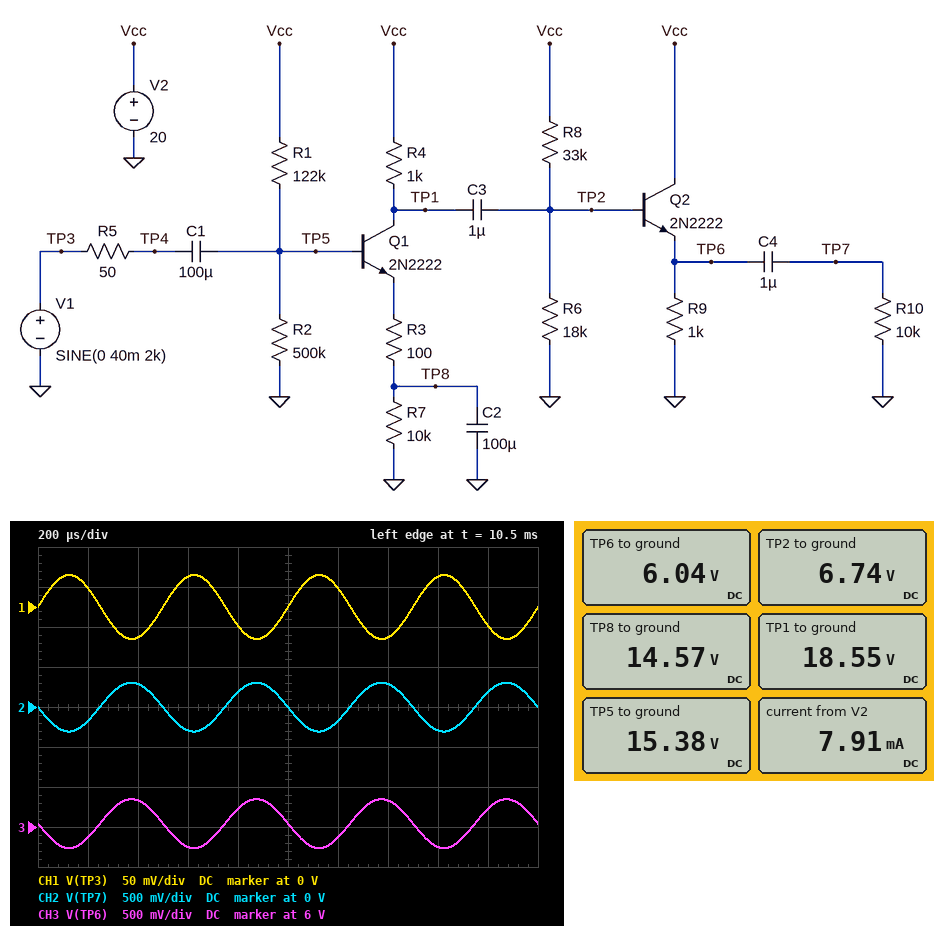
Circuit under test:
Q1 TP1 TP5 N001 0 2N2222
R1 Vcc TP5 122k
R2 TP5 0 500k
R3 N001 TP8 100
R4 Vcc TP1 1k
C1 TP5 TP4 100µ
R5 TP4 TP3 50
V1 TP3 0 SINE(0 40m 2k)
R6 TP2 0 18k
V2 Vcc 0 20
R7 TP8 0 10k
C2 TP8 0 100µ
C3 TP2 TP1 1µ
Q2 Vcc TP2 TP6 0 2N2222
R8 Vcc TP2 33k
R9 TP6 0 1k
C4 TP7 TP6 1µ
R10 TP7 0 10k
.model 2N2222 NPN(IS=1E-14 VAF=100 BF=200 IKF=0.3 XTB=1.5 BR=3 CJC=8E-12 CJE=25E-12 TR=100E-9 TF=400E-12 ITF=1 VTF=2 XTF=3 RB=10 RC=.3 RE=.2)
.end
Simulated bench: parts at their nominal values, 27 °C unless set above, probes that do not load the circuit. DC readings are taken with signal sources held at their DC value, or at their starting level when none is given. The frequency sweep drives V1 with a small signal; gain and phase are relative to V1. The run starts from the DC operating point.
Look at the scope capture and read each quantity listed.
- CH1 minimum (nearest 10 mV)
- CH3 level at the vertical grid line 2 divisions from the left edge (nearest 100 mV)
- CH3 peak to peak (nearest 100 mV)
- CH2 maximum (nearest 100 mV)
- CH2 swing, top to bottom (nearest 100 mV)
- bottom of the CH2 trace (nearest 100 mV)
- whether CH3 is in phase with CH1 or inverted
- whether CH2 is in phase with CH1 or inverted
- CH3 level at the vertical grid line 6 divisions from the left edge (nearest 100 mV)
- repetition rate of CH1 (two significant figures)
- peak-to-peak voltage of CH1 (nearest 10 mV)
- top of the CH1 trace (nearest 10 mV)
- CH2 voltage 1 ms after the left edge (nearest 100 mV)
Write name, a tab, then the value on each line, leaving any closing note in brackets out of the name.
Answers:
CH1 minimum	-40 mV
CH3 level at the vertical grid line 2 divisions from the left edge	6.3 V
CH3 peak to peak	600 mV
CH2 maximum	300 mV
CH2 swing, top to bottom	600 mV
bottom of the CH2 trace	-300 mV
whether CH3 is in phase with CH1 or inverted	inverted
whether CH2 is in phase with CH1 or inverted	inverted
CH3 level at the vertical grid line 6 divisions from the left edge	5.9 V
repetition rate of CH1	2.0 kHz
peak-to-peak voltage of CH1	80 mV
top of the CH1 trace	40 mV
CH2 voltage 1 ms after the left edge	0 V
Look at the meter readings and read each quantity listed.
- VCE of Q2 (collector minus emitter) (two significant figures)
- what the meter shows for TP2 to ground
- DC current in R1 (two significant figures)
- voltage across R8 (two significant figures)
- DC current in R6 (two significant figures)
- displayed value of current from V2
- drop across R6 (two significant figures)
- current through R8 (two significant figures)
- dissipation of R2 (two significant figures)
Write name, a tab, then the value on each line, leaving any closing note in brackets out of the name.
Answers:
VCE of Q2 (collector minus emitter)	14 V
what the meter shows for TP2 to ground	6.74 V
DC current in R1	38 µA
voltage across R8	13 V
DC current in R6	370 µA
displayed value of current from V2	7.91 mA
drop across R6	6.7 V
current through R8	400 µA
dissipation of R2	470 µW
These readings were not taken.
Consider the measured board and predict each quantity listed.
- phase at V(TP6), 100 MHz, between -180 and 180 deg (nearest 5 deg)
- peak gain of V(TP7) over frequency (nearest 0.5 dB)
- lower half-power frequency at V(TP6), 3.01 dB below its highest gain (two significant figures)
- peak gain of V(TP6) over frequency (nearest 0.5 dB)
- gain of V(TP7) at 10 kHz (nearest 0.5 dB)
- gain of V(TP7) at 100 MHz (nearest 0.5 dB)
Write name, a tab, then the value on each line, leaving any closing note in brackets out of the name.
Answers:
phase at V(TP6), 100 MHz, between -180 and 180 deg	45 deg
peak gain of V(TP7) over frequency	17.5 dB
lower half-power frequency at V(TP6), 3.01 dB below its highest gain	21 Hz
peak gain of V(TP6) over frequency	17.5 dB
gain of V(TP7) at 10 kHz	17.5 dB
gain of V(TP7) at 100 MHz	1.5 dB
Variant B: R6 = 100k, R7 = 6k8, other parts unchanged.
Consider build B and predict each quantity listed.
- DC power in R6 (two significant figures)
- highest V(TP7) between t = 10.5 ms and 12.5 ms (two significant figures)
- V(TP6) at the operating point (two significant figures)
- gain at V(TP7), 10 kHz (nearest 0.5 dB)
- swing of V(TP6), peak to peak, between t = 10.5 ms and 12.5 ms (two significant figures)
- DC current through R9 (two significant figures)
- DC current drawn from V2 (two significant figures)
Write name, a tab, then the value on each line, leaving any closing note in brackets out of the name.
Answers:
DC power in R6	1.8 mW
highest V(TP7) between t = 10.5 ms and 12.5 ms	330 mV
V(TP6) at the operating point	13 V
gain at V(TP7), 10 kHz	18.5 dB
swing of V(TP6), peak to peak, between t = 10.5 ms and 12.5 ms	670 mV
DC current through R9	13 mA
DC current drawn from V2	15 mA
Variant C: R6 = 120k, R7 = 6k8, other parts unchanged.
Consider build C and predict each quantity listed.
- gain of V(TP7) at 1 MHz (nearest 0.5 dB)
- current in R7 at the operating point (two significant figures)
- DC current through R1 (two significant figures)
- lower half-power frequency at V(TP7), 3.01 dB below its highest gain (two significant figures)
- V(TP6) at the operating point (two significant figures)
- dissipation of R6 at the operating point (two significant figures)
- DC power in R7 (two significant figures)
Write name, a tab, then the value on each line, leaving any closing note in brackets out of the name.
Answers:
gain of V(TP7) at 1 MHz	18.5 dB
current in R7 at the operating point	2.1 mA
DC current through R1	40 µA
lower half-power frequency at V(TP7), 3.01 dB below its highest gain	25 Hz
V(TP6) at the operating point	13 V
dissipation of R6 at the operating point	1.6 mW
DC power in R7	30 mW
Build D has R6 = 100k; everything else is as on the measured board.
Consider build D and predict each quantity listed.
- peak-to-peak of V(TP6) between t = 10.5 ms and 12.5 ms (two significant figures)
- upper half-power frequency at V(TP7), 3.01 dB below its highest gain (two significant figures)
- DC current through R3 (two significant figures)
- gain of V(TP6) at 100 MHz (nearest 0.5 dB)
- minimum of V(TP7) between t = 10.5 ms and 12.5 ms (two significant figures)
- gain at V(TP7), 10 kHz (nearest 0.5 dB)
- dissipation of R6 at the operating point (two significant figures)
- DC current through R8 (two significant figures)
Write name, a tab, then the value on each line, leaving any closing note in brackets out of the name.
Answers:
peak-to-peak of V(TP6) between t = 10.5 ms and 12.5 ms	640 mV
upper half-power frequency at V(TP7), 3.01 dB below its highest gain	14 MHz
DC current through R3	1.5 mA
gain of V(TP6) at 100 MHz	1.0 dB
minimum of V(TP7) between t = 10.5 ms and 12.5 ms	-320 mV
gain at V(TP7), 10 kHz	18.0 dB
dissipation of R6 at the operating point	1.8 mW
DC current through R8	200 µA
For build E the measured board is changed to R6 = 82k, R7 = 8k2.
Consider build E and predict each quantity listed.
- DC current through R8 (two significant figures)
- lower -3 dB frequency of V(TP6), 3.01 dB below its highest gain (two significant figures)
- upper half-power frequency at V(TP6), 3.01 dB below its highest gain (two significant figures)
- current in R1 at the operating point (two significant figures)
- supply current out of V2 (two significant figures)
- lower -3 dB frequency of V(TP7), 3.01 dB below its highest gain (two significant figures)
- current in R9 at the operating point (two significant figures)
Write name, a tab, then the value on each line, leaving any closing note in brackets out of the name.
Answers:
DC current through R8	220 µA
lower -3 dB frequency of V(TP6), 3.01 dB below its highest gain	17 Hz
upper half-power frequency at V(TP6), 3.01 dB below its highest gain	14 MHz
current in R1 at the operating point	39 µA
supply current out of V2	14 mA
lower -3 dB frequency of V(TP7), 3.01 dB below its highest gain	25 Hz
current in R9 at the operating point	12 mA
